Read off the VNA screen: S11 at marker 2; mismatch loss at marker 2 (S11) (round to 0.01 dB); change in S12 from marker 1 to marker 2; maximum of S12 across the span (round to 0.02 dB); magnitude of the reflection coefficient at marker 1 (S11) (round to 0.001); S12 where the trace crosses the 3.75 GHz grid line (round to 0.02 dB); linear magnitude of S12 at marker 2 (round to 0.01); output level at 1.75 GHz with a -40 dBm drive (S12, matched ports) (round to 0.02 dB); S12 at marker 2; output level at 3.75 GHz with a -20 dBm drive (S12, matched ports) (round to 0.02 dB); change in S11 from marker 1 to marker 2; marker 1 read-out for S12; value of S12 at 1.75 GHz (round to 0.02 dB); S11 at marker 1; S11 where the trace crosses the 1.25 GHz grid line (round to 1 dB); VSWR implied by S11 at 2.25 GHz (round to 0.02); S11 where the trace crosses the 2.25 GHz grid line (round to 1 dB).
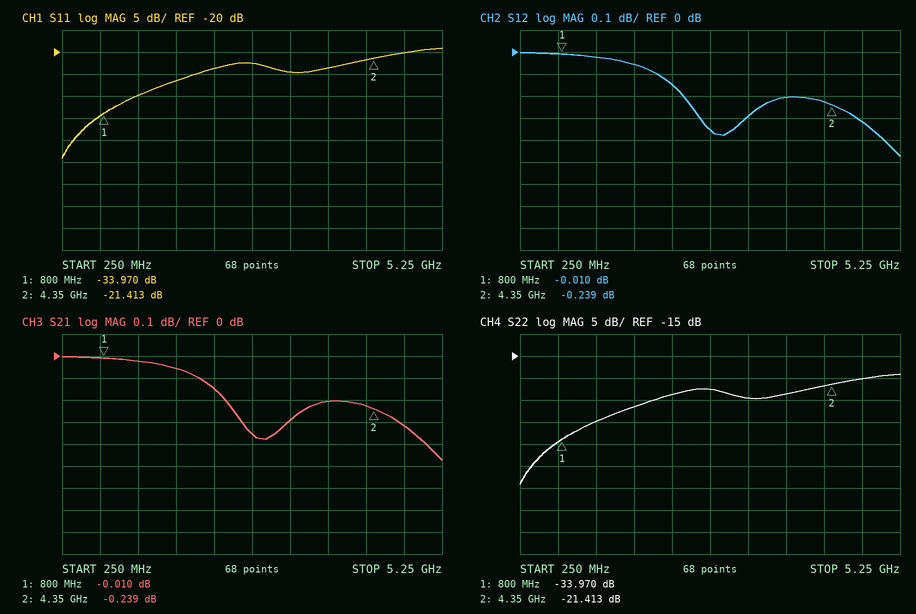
-21.413 dB
0.03 dB
-0.229 dB
0.00 dB
0.020
-0.20 dB
0.97
-40.06 dBm
-0.239 dB
-20.20 dBm
12.557 dB
-0.010 dB
-0.06 dB
-33.970 dB
-30 dB
1.14
-24 dB
